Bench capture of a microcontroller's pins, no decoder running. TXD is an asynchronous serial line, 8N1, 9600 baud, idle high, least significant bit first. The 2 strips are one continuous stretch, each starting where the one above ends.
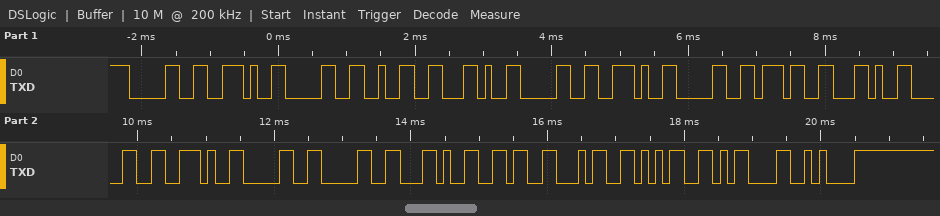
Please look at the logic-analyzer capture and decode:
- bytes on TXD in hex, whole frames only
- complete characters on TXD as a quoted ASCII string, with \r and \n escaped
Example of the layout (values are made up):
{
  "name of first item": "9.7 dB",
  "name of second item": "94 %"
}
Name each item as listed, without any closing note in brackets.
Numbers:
{
  "bytes on TXD in hex, whole frames only": "30 2E 30 32 2C 30 2E 30 37 2C 30 2E 30 30 2C 36 34 35 0D 0A",
  "complete characters on TXD as a quoted ASCII string, with \\r and \\n escaped": "\"0.02,0.07,0.00,645\\r\\n\""
}
